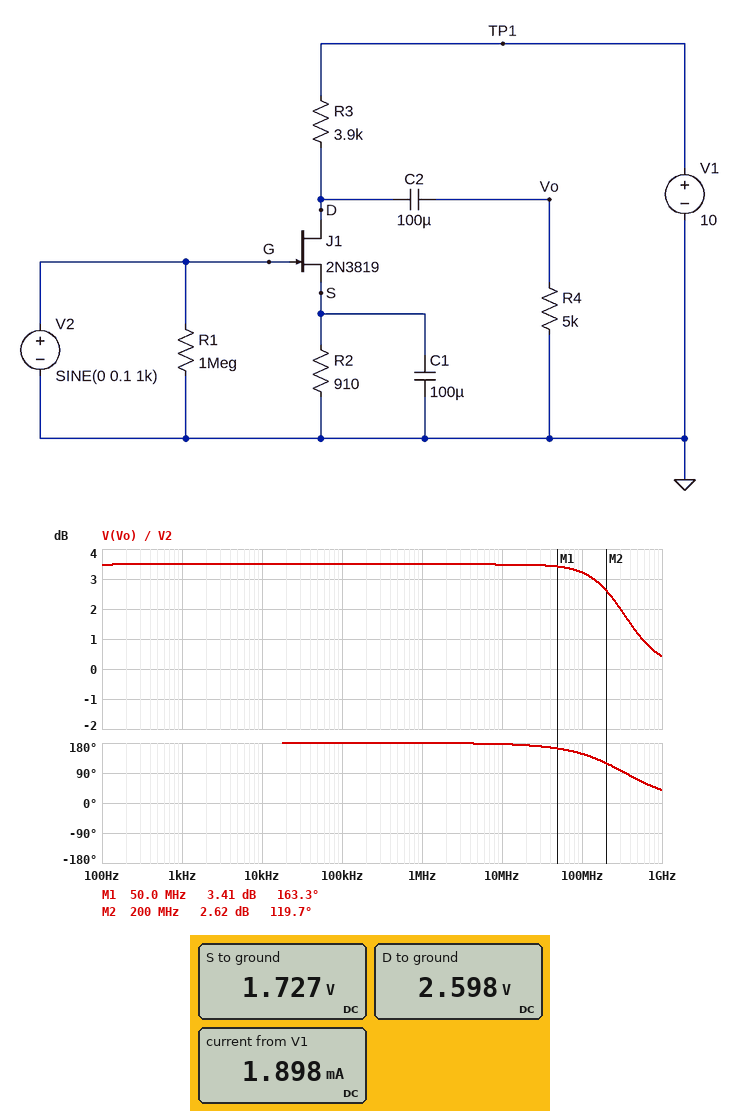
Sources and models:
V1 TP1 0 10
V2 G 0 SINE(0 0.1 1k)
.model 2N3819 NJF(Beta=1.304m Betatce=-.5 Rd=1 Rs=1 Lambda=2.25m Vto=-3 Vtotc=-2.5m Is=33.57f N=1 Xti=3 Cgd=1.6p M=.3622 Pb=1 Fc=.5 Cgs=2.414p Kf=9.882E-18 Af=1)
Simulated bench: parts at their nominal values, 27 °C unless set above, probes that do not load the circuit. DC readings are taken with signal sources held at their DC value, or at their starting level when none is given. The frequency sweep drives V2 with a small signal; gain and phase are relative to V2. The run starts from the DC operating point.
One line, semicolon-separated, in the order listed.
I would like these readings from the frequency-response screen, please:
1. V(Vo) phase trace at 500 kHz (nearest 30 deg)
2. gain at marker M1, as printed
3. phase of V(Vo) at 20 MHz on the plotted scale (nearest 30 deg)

180 deg; 3.41 dB; 180 deg
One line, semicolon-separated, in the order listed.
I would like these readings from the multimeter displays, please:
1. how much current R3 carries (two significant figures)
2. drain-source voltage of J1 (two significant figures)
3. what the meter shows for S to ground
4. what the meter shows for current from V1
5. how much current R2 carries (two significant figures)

1.9 mA; 870 mV; 1.727 V; 1.898 mA; 1.9 mA
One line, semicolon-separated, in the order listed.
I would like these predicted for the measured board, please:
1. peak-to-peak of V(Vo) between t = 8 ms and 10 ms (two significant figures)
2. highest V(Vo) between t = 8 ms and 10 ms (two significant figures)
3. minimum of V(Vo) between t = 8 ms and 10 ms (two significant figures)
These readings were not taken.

360 mV; 240 mV; -120 mV
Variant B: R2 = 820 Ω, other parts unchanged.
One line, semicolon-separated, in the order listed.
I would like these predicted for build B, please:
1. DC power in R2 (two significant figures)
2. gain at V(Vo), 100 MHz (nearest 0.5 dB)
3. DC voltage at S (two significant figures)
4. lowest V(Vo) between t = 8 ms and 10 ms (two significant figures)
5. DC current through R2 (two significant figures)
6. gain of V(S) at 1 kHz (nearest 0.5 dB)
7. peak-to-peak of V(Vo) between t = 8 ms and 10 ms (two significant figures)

3.2 mW; -1.0 dB; 1.6 V; -76 mV; 2.0 mA; -64.0 dB; 180 mV
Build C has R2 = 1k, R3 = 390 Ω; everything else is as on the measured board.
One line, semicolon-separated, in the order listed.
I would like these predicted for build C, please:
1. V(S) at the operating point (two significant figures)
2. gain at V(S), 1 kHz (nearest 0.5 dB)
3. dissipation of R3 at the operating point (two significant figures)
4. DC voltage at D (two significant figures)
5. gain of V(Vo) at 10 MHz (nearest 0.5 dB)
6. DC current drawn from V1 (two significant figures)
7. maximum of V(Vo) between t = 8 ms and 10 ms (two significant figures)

1.8 V; -46.0 dB; 1.3 mW; 9.3 V; 1.0 dB; 1.8 mA; 110 mV
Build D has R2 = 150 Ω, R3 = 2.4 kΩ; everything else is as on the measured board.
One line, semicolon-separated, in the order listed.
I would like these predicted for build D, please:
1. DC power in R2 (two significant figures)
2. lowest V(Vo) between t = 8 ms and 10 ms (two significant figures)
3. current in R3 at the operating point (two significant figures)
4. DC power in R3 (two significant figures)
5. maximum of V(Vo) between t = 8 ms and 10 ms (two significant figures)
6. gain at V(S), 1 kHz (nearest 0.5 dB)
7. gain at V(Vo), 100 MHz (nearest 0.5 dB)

2.0 mW; -31 mV; 3.7 mA; 32 mW; 35 mV; -70.0 dB; -9.0 dB
